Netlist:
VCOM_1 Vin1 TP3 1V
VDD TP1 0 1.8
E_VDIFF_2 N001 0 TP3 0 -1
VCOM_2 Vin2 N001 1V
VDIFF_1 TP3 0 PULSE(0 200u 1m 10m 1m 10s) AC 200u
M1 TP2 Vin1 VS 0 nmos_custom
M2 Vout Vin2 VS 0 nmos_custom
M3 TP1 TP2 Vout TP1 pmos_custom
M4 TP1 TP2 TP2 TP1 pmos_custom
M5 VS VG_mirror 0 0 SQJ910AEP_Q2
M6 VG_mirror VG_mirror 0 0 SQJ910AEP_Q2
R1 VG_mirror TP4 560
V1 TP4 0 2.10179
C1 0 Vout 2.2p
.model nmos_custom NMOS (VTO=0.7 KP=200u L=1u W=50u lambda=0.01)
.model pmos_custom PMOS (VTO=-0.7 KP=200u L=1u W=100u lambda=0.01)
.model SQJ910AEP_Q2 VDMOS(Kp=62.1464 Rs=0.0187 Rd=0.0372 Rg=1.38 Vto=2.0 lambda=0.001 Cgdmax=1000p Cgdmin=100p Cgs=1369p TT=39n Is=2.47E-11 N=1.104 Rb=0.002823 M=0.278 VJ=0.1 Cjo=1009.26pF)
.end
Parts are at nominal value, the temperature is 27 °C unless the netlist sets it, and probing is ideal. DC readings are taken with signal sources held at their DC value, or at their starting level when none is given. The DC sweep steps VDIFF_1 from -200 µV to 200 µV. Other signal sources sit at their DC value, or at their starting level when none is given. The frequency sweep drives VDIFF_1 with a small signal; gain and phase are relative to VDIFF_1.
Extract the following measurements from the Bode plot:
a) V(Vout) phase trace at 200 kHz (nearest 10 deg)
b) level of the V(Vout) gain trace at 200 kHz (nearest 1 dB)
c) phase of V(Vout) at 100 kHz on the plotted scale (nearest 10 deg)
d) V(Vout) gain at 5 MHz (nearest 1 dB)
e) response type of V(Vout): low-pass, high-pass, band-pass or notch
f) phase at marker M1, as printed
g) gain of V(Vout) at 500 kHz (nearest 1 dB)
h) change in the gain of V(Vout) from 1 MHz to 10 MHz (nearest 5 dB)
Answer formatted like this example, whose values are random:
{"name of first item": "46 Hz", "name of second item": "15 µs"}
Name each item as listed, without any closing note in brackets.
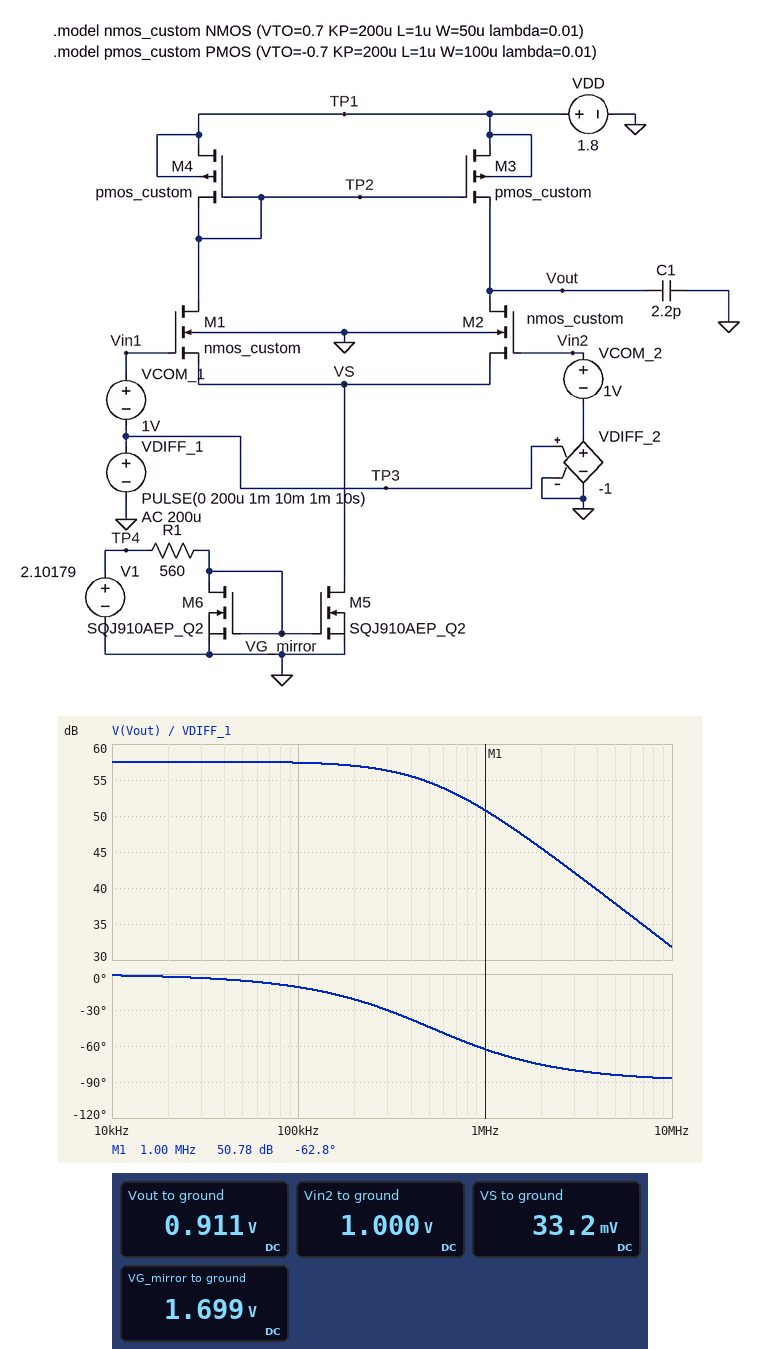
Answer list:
{"V(Vout) phase trace at 200 kHz": "-20 deg", "level of the V(Vout) gain trace at 200 kHz": "57 dB", "phase of V(Vout) at 100 kHz on the plotted scale": "-10 deg", "V(Vout) gain at 5 MHz": "38 dB", "response type of V(Vout): low-pass, high-pass, band-pass or notch": "low-pass", "phase at marker M1, as printed": "-62.8 deg", "gain of V(Vout) at 500 kHz": "55 dB", "change in the gain of V(Vout) from 1 MHz to 10 MHz": "-20 dB"}
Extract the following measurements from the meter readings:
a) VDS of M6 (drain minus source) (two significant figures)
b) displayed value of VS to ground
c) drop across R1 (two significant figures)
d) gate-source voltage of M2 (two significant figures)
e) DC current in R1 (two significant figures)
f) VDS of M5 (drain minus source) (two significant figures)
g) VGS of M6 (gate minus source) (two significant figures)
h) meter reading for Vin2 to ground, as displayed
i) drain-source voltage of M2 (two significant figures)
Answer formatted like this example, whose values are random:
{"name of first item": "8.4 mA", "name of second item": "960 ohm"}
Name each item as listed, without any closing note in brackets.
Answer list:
{"VDS of M6 (drain minus source)": "1.7 V", "displayed value of VS to ground": "33.2 mV", "drop across R1": "400 mV", "gate-source voltage of M2": "970 mV", "DC current in R1": "720 µA", "VDS of M5 (drain minus source)": "33 mV", "VGS of M6 (gate minus source)": "1.7 V", "meter reading for Vin2 to ground, as displayed": "1.000 V", "drain-source voltage of M2": "880 mV"}
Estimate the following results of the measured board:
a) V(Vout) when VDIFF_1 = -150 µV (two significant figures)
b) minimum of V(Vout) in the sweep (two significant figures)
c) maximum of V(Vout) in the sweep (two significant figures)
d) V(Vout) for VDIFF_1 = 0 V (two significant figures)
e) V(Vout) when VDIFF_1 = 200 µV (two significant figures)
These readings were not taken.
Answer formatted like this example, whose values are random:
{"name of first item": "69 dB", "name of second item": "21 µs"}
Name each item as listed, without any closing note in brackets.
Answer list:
{"V(Vout) when VDIFF_1 = -150 µV": "800 mV", "minimum of V(Vout) in the sweep": "760 mV", "maximum of V(Vout) in the sweep": "1.1 V", "V(Vout) for VDIFF_1 = 0 V": "910 mV", "V(Vout) when VDIFF_1 = 200 µV": "1.1 V"}
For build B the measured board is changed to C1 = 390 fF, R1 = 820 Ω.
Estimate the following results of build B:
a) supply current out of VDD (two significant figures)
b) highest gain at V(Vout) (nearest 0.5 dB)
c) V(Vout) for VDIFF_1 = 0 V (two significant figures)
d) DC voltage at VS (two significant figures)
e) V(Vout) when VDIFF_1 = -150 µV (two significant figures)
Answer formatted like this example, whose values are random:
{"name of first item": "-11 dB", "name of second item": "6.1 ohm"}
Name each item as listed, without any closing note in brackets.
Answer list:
{"supply current out of VDD": "510 µA", "highest gain at V(Vout)": "59.0 dB", "V(Vout) for VDIFF_1 = 0 V": "940 mV", "DC voltage at VS": "75 mV", "V(Vout) when VDIFF_1 = -150 µV": "810 mV"}
